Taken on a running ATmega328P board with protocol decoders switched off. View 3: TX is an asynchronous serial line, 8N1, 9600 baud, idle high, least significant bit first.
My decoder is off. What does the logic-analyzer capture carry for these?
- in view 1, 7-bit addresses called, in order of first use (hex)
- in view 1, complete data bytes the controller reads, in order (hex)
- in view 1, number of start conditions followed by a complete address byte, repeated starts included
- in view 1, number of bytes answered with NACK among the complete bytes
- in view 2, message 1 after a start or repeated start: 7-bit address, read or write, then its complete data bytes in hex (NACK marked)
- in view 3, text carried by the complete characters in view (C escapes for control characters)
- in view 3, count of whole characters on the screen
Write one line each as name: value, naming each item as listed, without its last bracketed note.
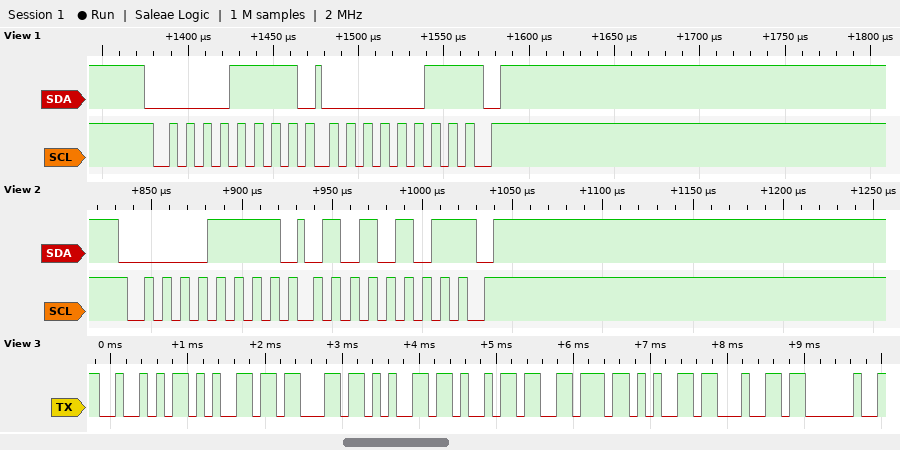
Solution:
in view 1, 7-bit addresses called, in order of first use: 0x07
in view 1, complete data bytes the controller reads, in order: 03
in view 1, number of start conditions followed by a complete address byte, repeated starts included: 1
in view 1, number of bytes answered with NACK among the complete bytes: 1
in view 2, message 1 after a start or repeated start: 7-bit address, read or write, then its complete data bytes in hex: 0x07 read: 55 NACK
in view 3, text carried by the complete characters in view: "Received "
in view 3, count of whole characters on the screen: 9
